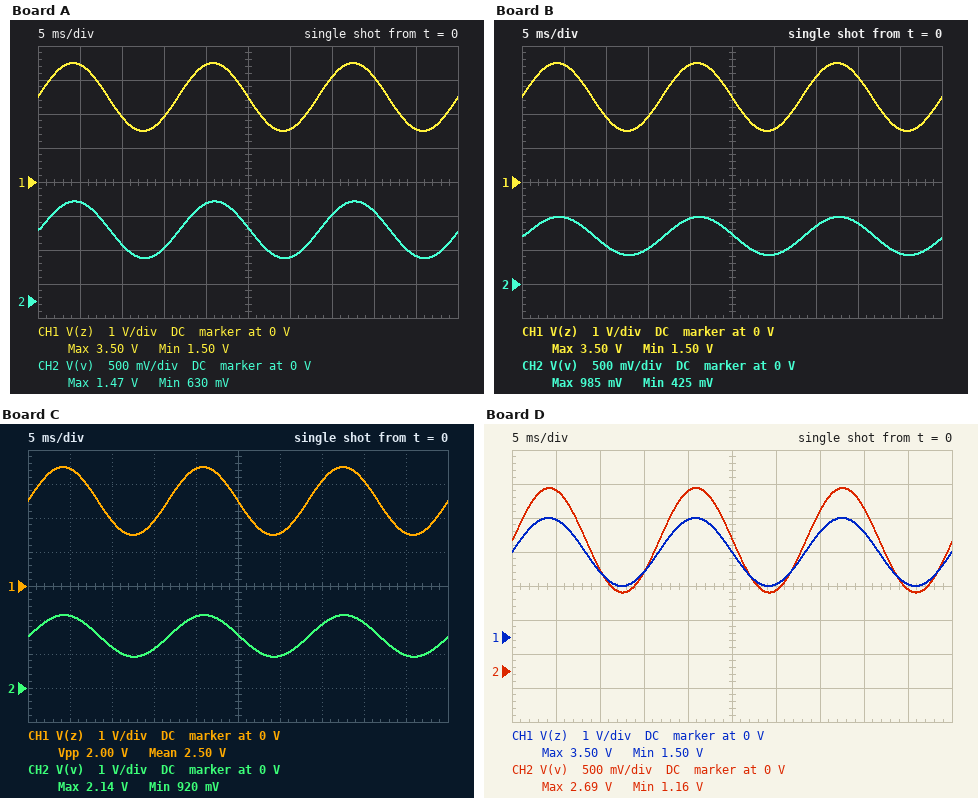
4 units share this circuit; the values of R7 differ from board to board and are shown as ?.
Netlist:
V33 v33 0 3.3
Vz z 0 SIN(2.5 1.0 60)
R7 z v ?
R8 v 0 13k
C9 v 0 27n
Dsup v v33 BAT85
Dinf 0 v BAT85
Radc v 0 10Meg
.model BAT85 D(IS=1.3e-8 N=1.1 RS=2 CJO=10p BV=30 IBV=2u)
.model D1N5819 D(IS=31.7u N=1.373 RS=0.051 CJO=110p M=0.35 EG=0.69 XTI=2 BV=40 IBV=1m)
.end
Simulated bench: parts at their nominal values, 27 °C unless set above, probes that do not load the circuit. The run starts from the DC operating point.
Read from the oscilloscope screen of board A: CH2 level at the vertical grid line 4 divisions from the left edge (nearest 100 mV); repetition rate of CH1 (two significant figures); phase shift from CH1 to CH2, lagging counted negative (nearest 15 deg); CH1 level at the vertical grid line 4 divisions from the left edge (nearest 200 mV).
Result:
1.4 V
60 Hz
0 deg
3.4 V
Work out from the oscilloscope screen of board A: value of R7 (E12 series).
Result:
18 kΩ
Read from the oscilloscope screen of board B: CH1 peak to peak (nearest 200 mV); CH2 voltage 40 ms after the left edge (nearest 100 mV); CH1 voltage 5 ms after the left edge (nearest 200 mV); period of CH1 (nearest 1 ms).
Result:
2.0 V
900 mV
3.4 V
17 ms
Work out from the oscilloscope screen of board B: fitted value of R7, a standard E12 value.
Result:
33 kΩ
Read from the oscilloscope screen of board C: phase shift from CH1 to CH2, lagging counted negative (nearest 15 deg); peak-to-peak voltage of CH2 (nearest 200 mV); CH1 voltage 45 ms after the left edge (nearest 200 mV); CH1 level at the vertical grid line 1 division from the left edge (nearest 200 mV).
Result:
0 deg
1.2 V
1.6 V
3.4 V
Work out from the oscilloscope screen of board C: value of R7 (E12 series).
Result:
8.2 kΩ
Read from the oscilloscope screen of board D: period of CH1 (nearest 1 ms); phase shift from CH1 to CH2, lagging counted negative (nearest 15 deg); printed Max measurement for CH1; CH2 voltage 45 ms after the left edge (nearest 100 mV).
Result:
17 ms
0 deg
3.50 V
1.2 V
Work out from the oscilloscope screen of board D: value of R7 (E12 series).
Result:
3.9 kΩ
